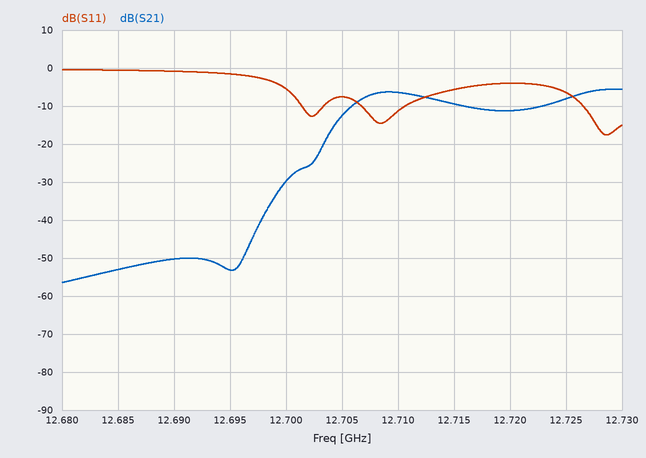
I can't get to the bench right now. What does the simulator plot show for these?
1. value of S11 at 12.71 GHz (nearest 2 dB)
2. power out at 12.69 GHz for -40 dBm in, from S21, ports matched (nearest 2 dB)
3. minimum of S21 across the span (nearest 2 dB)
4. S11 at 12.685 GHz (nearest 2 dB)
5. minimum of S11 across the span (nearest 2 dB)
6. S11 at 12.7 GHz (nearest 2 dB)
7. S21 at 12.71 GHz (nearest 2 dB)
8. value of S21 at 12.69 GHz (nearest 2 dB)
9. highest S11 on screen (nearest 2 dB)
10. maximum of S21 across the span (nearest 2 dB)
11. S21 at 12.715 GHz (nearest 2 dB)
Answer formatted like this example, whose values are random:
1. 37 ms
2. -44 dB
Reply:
1. -12 dB
2. -90 dBm
3. -56 dB
4. 0 dB
5. -18 dB
6. -6 dB
7. -6 dB
8. -50 dB
9. 0 dB
10. -6 dB
11. -10 dB
